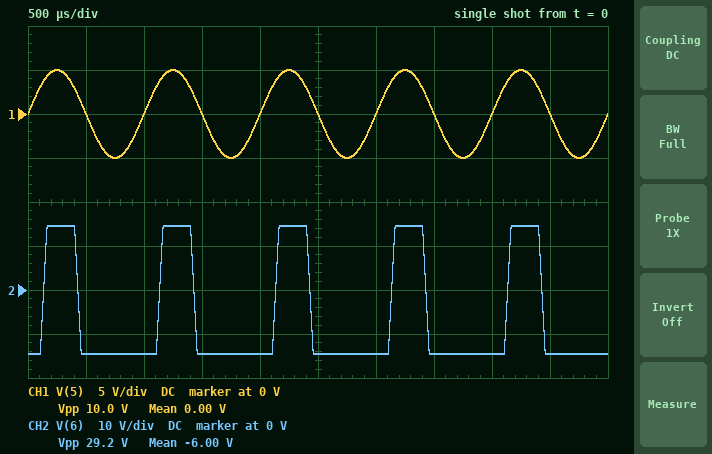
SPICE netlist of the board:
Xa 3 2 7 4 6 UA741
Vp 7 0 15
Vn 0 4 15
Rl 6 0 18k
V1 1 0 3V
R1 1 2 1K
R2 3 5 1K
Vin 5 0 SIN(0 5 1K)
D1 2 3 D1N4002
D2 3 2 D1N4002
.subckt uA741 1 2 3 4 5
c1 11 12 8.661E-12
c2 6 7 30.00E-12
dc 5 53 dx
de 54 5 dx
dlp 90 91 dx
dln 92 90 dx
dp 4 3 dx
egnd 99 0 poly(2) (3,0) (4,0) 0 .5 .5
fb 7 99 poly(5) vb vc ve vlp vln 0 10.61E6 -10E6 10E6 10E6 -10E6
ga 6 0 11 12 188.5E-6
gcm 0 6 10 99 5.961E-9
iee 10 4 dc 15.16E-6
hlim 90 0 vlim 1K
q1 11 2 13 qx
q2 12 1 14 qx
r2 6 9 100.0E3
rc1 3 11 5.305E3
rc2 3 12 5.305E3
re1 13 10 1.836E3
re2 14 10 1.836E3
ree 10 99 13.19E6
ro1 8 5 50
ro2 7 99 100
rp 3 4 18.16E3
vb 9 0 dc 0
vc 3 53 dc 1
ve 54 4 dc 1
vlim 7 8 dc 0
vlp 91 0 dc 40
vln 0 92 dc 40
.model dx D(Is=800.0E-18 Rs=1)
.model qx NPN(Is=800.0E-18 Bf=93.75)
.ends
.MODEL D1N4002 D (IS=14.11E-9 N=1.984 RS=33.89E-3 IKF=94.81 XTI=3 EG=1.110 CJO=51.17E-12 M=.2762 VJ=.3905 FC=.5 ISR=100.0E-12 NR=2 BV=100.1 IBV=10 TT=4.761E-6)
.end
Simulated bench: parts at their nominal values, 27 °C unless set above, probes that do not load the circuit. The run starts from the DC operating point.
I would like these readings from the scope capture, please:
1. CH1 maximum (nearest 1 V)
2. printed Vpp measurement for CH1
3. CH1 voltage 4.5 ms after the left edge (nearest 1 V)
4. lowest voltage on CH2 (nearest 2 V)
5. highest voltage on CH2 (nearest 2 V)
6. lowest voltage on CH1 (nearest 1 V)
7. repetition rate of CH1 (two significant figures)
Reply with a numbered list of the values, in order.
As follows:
1. 5 V
2. 10.0 V
3. 0 V
4. -14 V
5. 14 V
6. -5 V
7. 1.0 kHz
